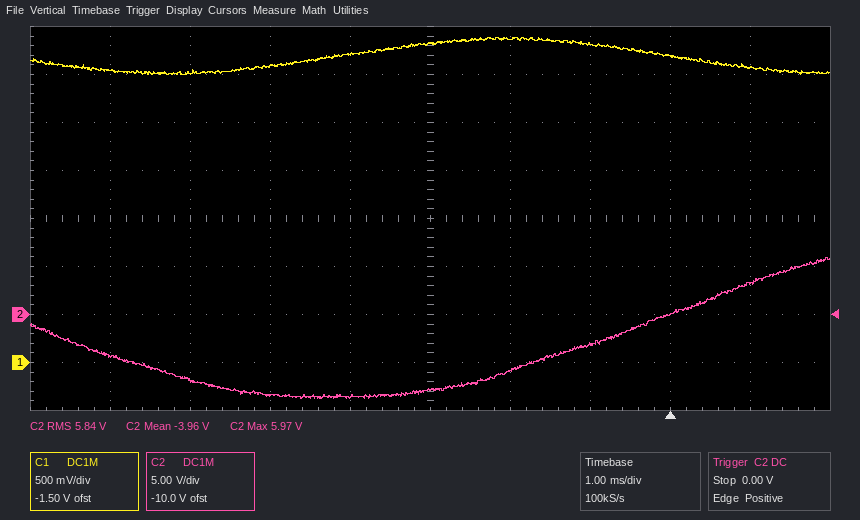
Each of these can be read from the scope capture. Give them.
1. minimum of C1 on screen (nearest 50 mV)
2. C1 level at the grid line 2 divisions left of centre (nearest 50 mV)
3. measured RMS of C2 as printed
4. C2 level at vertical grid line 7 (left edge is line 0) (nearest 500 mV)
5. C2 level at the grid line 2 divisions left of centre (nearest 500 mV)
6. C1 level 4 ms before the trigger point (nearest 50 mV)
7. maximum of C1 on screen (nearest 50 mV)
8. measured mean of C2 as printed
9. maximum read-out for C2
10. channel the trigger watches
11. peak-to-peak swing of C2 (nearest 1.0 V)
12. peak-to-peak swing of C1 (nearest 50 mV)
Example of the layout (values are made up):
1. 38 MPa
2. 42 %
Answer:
1. 3.00 V
2. 3.10 V
3. 5.84 V
4. -3.0 V
5. -8.5 V
6. 3.20 V
7. 3.40 V
8. -3.96 V
9. 5.97 V
10. C2
11. 15.0 V
12. 400 mV
